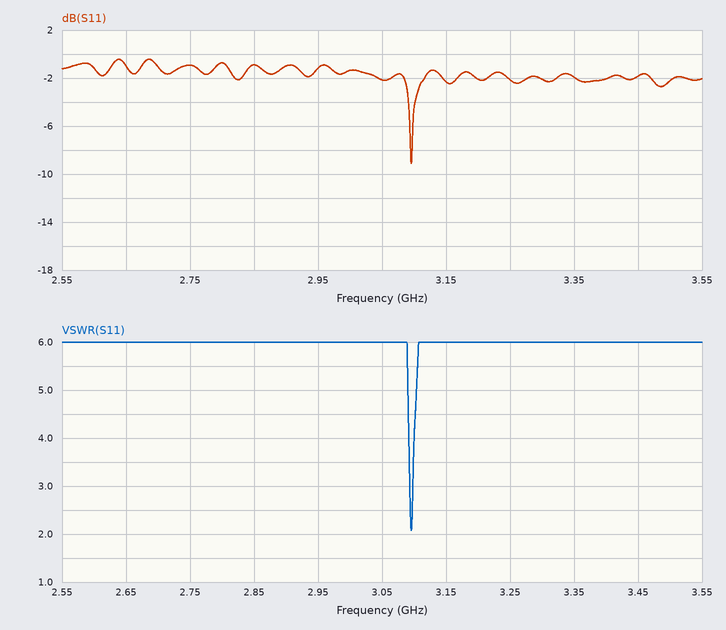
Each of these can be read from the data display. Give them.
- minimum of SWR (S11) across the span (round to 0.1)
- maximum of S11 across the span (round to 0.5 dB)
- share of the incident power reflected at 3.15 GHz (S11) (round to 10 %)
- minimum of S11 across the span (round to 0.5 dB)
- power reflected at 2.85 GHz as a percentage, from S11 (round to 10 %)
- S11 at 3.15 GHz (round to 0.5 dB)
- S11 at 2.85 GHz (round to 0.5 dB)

2.1
-0.5 dB
60 %
-9.0 dB
80 %
-2.5 dB
-1.0 dB
